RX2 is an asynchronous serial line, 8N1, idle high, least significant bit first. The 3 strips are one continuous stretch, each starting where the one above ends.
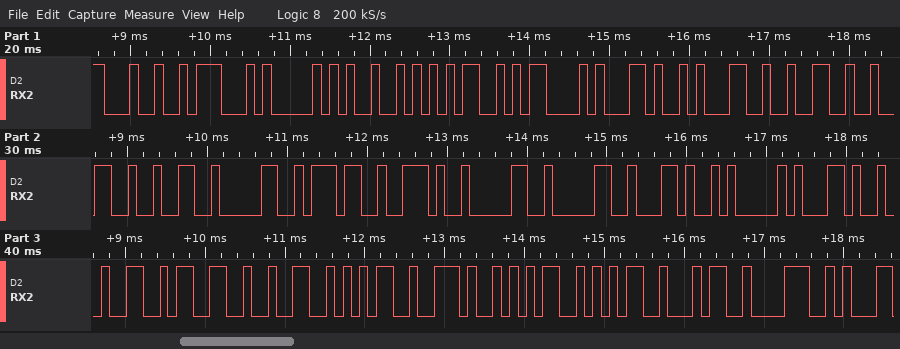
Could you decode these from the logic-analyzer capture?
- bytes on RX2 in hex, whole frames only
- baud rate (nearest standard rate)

0x24 0x47 0x50 0x52 0x4D 0x43 0x2C 0x31 0x32 0x32 0x32 0x30 0x37 0x2E 0x30 0x30 0x2C 0x41 0x2C 0x32 0x33 0x32 0x35 0x2E 0x35 0x35 0x34 0x38
9600 baud
